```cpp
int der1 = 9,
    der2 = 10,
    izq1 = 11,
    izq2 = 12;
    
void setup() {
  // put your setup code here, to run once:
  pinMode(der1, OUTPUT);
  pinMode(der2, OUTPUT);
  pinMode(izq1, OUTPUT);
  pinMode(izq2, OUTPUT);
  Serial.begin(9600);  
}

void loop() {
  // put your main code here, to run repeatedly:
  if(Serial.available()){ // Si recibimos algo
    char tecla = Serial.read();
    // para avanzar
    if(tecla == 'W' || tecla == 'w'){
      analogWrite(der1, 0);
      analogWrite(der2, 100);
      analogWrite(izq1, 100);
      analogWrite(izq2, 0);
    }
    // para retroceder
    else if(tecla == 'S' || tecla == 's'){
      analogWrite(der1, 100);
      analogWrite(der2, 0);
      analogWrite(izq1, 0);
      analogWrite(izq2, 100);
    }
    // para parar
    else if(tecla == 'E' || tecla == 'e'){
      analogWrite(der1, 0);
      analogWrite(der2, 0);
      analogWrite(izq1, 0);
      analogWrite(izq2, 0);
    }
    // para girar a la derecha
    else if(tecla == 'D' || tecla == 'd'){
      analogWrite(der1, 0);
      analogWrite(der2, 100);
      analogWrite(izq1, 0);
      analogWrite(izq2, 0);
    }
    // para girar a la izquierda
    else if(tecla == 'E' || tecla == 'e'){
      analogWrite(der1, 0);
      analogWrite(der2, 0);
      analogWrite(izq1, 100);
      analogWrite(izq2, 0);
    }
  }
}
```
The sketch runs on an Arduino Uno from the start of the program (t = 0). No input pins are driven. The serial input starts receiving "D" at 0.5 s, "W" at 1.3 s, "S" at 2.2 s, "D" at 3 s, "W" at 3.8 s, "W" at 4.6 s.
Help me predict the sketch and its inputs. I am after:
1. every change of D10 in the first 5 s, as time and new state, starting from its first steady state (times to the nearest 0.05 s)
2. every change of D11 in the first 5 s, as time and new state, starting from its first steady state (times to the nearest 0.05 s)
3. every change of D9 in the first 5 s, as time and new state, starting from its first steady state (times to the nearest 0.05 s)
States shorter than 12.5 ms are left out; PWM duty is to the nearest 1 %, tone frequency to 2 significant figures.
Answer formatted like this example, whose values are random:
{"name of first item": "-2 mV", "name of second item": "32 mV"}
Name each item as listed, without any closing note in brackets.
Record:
{"every change of D10 in the first 5 s, as time and new state, starting from its first steady state": "0 s low; 0.5 s PWM 39 %; 2.2 s low; 3 s PWM 39 %", "every change of D11 in the first 5 s, as time and new state, starting from its first steady state": "0 s low; 1.3 s PWM 39 %; 2.2 s low; 3.8 s PWM 39 %", "every change of D9 in the first 5 s, as time and new state, starting from its first steady state": "0 s low; 2.2 s PWM 39 %; 3 s low"}
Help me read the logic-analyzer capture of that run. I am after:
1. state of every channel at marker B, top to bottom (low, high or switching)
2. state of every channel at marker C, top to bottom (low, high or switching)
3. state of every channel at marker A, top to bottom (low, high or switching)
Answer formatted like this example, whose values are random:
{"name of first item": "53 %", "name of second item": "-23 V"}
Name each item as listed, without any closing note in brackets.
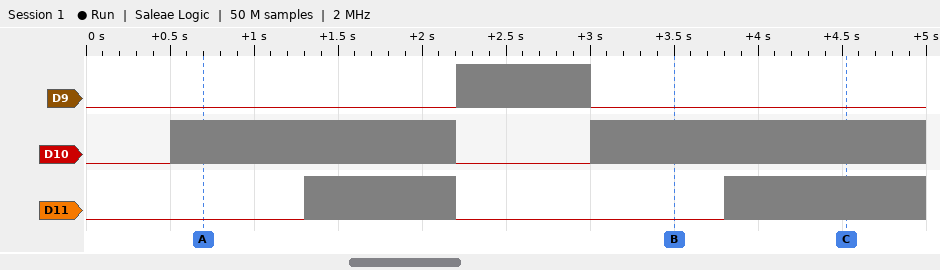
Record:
{"state of every channel at marker B, top to bottom": "D9 low, D10 switching, D11 low", "state of every channel at marker C, top to bottom": "D9 low, D10 switching, D11 switching", "state of every channel at marker A, top to bottom": "D9 low, D10 switching, D11 low"}
